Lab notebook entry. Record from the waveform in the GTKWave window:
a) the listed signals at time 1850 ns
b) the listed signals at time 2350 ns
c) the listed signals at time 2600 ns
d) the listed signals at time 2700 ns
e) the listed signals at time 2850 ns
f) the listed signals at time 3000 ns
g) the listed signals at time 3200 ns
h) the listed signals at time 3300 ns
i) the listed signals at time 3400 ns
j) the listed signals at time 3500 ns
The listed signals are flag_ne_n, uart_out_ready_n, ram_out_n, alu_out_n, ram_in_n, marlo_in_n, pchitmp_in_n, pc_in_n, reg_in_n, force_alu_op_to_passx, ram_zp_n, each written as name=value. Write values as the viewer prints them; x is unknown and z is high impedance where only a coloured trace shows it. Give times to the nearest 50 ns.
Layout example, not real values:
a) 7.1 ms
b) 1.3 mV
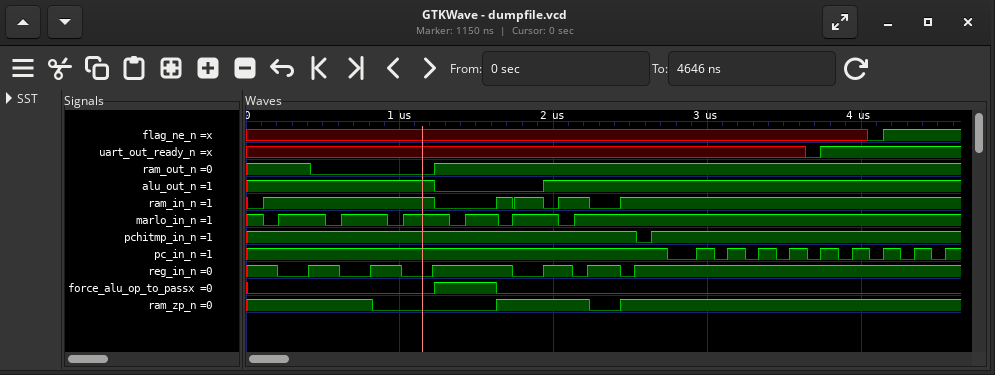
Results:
a) flag_ne_n=x, uart_out_ready_n=x, ram_out_n=1, alu_out_n=0, ram_in_n=1, marlo_in_n=1, pchitmp_in_n=1, pc_in_n=1, reg_in_n=0, force_alu_op_to_passx=0, ram_zp_n=1
b) flag_ne_n=x, uart_out_ready_n=x, ram_out_n=1, alu_out_n=1, ram_in_n=0, marlo_in_n=1, pchitmp_in_n=1, pc_in_n=1, reg_in_n=1, force_alu_op_to_passx=0, ram_zp_n=0
c) flag_ne_n=x, uart_out_ready_n=x, ram_out_n=1, alu_out_n=1, ram_in_n=1, marlo_in_n=1, pchitmp_in_n=0, pc_in_n=1, reg_in_n=1, force_alu_op_to_passx=0, ram_zp_n=1
d) flag_ne_n=x, uart_out_ready_n=x, ram_out_n=1, alu_out_n=1, ram_in_n=1, marlo_in_n=1, pchitmp_in_n=1, pc_in_n=1, reg_in_n=1, force_alu_op_to_passx=0, ram_zp_n=1
e) flag_ne_n=x, uart_out_ready_n=x, ram_out_n=1, alu_out_n=1, ram_in_n=1, marlo_in_n=1, pchitmp_in_n=1, pc_in_n=0, reg_in_n=1, force_alu_op_to_passx=0, ram_zp_n=1
f) flag_ne_n=x, uart_out_ready_n=x, ram_out_n=1, alu_out_n=1, ram_in_n=1, marlo_in_n=1, pchitmp_in_n=1, pc_in_n=1, reg_in_n=1, force_alu_op_to_passx=0, ram_zp_n=1
g) flag_ne_n=x, uart_out_ready_n=x, ram_out_n=1, alu_out_n=1, ram_in_n=1, marlo_in_n=1, pchitmp_in_n=1, pc_in_n=1, reg_in_n=1, force_alu_op_to_passx=0, ram_zp_n=1
h) flag_ne_n=x, uart_out_ready_n=x, ram_out_n=1, alu_out_n=1, ram_in_n=1, marlo_in_n=1, pchitmp_in_n=1, pc_in_n=0, reg_in_n=1, force_alu_op_to_passx=0, ram_zp_n=1
i) flag_ne_n=x, uart_out_ready_n=x, ram_out_n=1, alu_out_n=1, ram_in_n=1, marlo_in_n=1, pchitmp_in_n=1, pc_in_n=1, reg_in_n=1, force_alu_op_to_passx=0, ram_zp_n=1
j) flag_ne_n=x, uart_out_ready_n=x, ram_out_n=1, alu_out_n=1, ram_in_n=1, marlo_in_n=1, pchitmp_in_n=1, pc_in_n=0, reg_in_n=1, force_alu_op_to_passx=0, ram_zp_n=1
